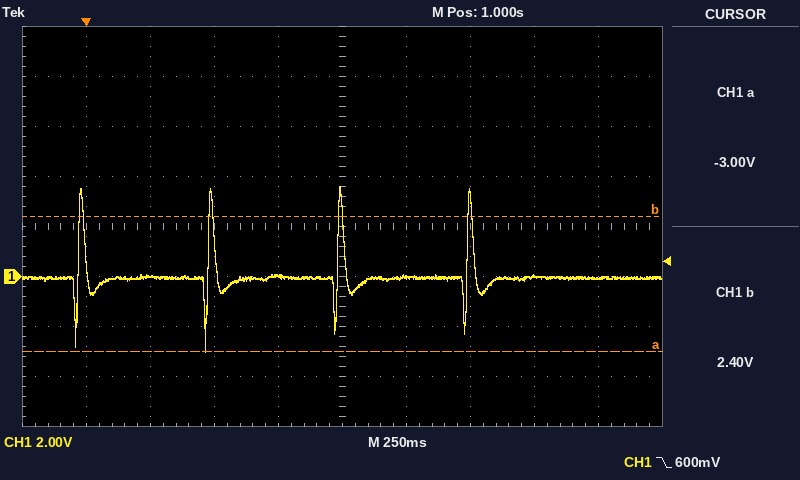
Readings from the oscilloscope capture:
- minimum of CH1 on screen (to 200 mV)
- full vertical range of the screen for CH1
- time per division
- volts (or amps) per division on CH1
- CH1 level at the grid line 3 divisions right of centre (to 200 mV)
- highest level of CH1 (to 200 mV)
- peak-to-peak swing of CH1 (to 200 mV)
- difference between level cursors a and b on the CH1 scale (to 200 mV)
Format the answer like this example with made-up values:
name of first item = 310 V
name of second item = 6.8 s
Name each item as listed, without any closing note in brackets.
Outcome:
minimum of CH1 on screen = -3.0 V
full vertical range of the screen for CH1 = 16 V
time per division = 250 ms
volts (or amps) per division on CH1 = 2 V
CH1 level at the grid line 3 divisions right of centre = 0.0 V
highest level of CH1 = 3.6 V
peak-to-peak swing of CH1 = 6.6 V
difference between level cursors a and b on the CH1 scale = 5.4 V
